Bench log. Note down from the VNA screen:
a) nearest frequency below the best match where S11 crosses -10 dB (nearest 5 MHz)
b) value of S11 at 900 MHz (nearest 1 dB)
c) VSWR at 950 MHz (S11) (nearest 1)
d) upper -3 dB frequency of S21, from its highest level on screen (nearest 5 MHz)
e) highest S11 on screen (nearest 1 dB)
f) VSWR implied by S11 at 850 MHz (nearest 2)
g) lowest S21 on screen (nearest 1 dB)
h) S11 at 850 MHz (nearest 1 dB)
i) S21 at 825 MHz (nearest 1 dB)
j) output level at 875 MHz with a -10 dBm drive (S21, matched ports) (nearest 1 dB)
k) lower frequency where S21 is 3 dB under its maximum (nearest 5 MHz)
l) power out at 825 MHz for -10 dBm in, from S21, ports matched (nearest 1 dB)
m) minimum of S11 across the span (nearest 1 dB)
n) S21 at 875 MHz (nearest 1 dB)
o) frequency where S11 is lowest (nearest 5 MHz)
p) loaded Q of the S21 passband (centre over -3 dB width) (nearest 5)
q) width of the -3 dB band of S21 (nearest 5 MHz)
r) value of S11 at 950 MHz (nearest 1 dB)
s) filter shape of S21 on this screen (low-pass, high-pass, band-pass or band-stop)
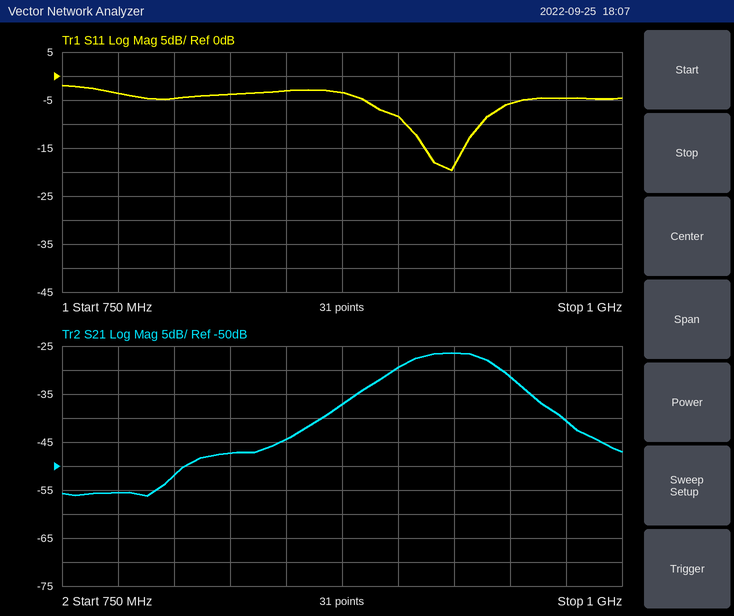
905 MHz
-8 dB
3
945 MHz
-2 dB
6
-56 dB
-3 dB
-47 dB
-47 dBm
900 MHz
-57 dBm
-20 dB
-37 dB
925 MHz
20
45 MHz
-6 dB
band-pass
